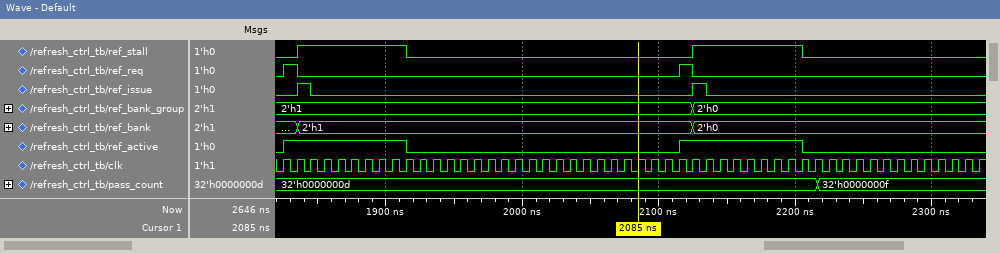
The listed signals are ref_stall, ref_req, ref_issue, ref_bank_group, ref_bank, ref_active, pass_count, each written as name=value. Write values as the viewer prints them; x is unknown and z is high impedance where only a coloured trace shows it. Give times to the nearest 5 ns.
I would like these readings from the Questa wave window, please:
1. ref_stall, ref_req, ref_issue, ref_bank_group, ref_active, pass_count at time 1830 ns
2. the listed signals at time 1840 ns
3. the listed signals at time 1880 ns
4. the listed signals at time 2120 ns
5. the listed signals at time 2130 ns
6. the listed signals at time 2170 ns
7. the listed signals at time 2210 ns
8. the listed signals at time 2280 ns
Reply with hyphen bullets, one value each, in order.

- ref_stall=0, ref_req=1, ref_issue=0, ref_bank_group=2'h1, ref_active=1, pass_count=32'h0000000d
- ref_stall=1, ref_req=0, ref_issue=1, ref_bank_group=2'h1, ref_bank=2'h1, ref_active=1, pass_count=32'h0000000d
- ref_stall=1, ref_req=0, ref_issue=0, ref_bank_group=2'h1, ref_bank=2'h1, ref_active=1, pass_count=32'h0000000d
- ref_stall=0, ref_req=1, ref_issue=0, ref_bank_group=2'h1, ref_bank=2'h1, ref_active=1, pass_count=32'h0000000d
- ref_stall=1, ref_req=0, ref_issue=1, ref_bank_group=2'h0, ref_bank=2'h0, ref_active=1, pass_count=32'h0000000d
- ref_stall=1, ref_req=0, ref_issue=0, ref_bank_group=2'h0, ref_bank=2'h0, ref_active=1, pass_count=32'h0000000d
- ref_stall=0, ref_req=0, ref_issue=0, ref_bank_group=2'h0, ref_bank=2'h0, ref_active=0, pass_count=32'h0000000d
- ref_stall=0, ref_req=0, ref_issue=0, ref_bank_group=2'h0, ref_bank=2'h0, ref_active=0, pass_count=32'h0000000f
